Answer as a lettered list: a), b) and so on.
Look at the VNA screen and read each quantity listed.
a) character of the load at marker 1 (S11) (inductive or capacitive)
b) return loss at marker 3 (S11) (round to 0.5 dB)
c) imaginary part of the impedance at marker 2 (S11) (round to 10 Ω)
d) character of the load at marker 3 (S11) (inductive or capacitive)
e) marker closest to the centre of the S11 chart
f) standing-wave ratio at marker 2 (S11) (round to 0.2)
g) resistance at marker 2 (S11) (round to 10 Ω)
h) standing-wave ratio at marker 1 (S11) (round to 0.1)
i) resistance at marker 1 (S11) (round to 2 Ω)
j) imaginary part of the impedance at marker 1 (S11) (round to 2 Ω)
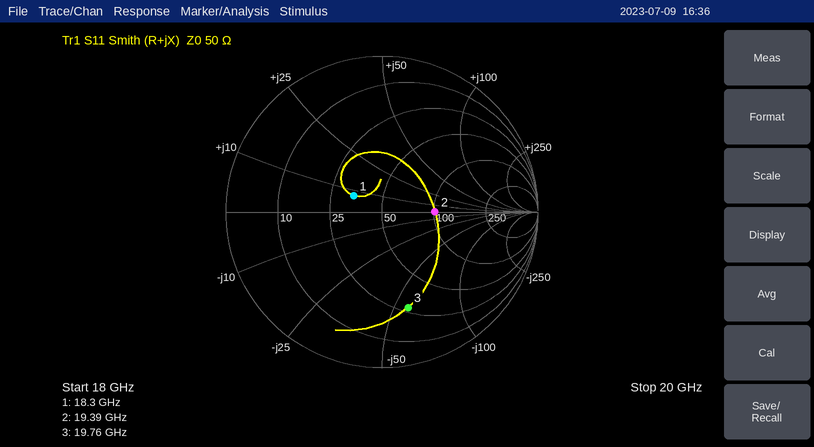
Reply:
a) inductive
b) 4.0 dB
c) 0 Ω
d) capacitive
e) marker 1
f) 2.0
g) 100 Ω
h) 1.5
i) 34 Ω
j) +8 Ω
